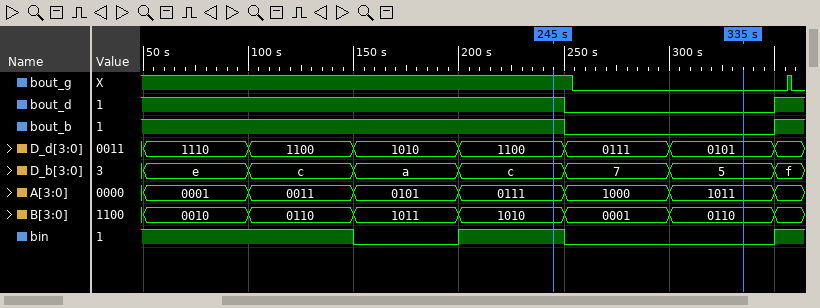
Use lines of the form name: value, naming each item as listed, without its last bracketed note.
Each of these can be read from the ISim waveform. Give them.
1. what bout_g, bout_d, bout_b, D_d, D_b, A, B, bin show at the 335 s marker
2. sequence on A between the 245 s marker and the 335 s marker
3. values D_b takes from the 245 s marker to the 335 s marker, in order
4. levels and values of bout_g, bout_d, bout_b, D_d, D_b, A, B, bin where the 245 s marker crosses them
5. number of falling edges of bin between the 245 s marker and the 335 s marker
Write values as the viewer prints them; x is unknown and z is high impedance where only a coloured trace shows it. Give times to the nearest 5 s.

what bout_g, bout_d, bout_b, D_d, D_b, A, B, bin show at the 335 s marker: bout_g=0, bout_d=0, bout_b=0, D_d=0101, D_b=5, A=1011, B=0110, bin=0
sequence on A between the 245 s marker and the 335 s marker: 0111, 1000, 1011
values D_b takes from the 245 s marker to the 335 s marker, in order: c, 7, 5
levels and values of bout_g, bout_d, bout_b, D_d, D_b, A, B, bin where the 245 s marker crosses them: bout_g=1, bout_d=1, bout_b=1, D_d=1100, D_b=c, A=0111, B=1010, bin=1
number of falling edges of bin between the 245 s marker and the 335 s marker: 1
